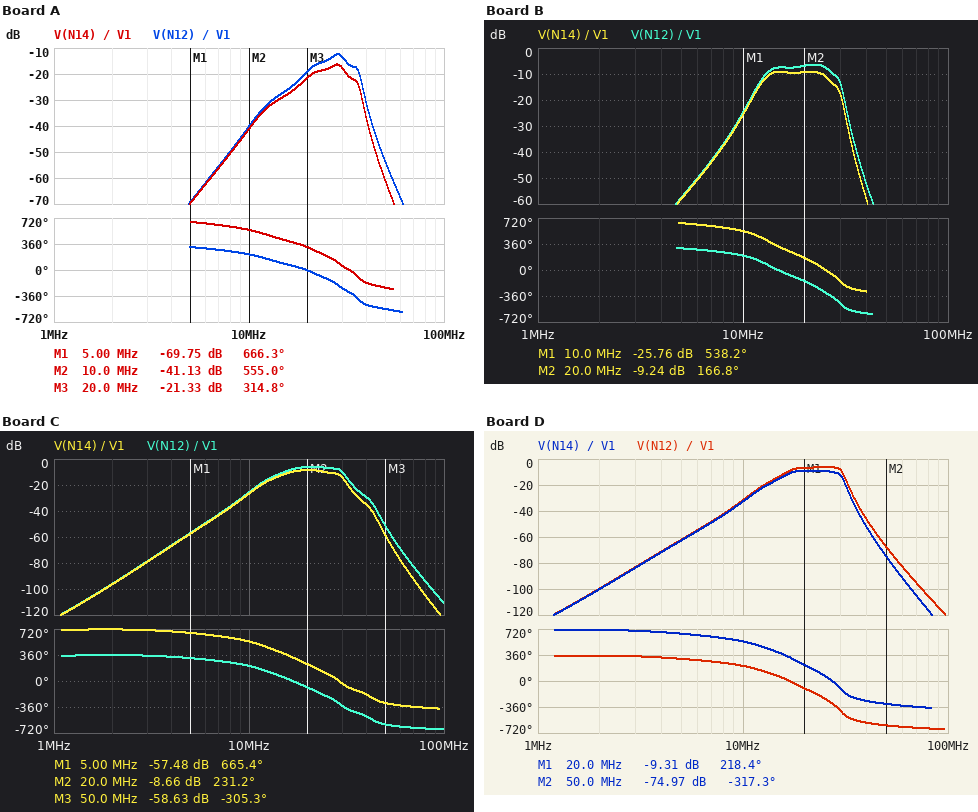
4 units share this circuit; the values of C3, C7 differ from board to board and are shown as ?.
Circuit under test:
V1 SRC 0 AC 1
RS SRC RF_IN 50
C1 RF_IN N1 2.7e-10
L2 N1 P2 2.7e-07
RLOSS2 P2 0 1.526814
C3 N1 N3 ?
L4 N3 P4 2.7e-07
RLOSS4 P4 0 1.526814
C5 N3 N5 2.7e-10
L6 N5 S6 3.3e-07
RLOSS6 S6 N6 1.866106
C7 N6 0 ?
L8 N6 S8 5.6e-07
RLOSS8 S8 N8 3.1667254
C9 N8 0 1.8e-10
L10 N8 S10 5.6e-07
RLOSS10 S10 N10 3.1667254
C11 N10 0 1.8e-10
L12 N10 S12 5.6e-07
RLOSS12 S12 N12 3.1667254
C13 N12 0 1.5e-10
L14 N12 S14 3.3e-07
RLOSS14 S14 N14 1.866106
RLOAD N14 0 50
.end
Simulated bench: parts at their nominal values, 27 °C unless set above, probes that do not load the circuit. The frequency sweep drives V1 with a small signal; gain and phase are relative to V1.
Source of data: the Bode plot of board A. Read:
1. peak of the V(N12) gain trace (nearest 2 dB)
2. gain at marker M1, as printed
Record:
-12 dB
-69.75 dB
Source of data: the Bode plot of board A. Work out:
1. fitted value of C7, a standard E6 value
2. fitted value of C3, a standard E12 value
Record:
68 pF
39 pF
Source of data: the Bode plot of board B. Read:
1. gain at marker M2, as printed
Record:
-9.24 dB
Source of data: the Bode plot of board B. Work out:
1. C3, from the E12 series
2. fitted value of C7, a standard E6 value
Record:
180 pF
330 pF
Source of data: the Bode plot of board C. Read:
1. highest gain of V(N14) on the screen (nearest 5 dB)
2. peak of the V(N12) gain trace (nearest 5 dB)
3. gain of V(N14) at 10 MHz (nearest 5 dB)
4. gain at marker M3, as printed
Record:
-10 dB
-5 dB
-25 dB
-58.63 dB
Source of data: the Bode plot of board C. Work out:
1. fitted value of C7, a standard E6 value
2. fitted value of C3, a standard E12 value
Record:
68 pF
150 pF
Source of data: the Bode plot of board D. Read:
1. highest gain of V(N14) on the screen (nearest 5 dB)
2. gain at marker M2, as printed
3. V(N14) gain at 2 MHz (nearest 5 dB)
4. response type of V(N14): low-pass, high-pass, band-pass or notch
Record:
-10 dB
-74.97 dB
-100 dB
band-pass
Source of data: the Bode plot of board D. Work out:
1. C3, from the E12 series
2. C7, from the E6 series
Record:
100 pF
220 pF
